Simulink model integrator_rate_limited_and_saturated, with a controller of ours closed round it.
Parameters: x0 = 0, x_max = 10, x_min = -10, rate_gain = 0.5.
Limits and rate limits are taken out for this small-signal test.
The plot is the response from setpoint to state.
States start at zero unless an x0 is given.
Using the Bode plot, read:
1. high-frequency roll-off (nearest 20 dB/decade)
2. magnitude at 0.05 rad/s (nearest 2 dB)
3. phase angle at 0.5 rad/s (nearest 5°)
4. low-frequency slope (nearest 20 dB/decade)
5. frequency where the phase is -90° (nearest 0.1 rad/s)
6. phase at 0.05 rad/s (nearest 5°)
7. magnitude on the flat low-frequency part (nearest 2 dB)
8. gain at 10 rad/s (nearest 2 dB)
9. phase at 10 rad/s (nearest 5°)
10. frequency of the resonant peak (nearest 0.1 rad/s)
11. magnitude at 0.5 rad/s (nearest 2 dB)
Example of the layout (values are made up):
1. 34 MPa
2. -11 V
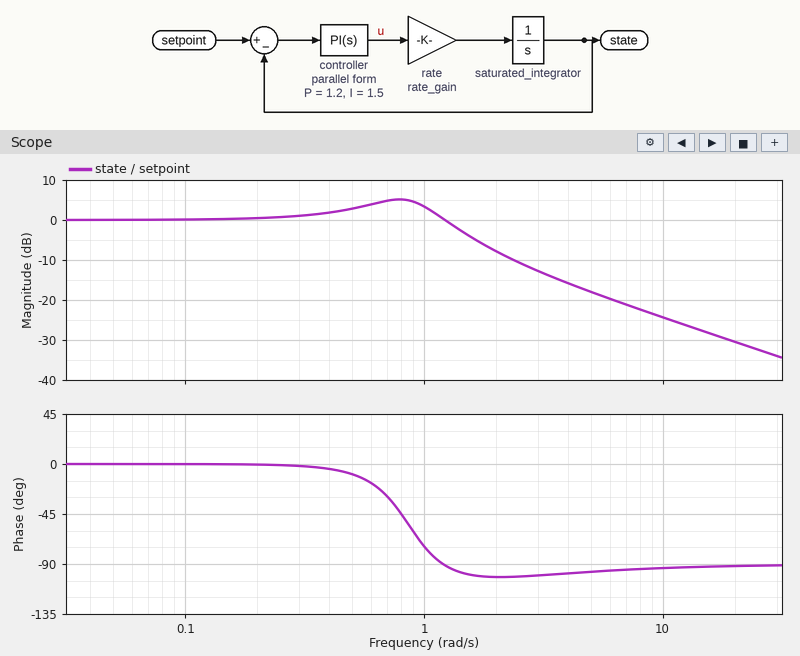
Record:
1. -20 dB/decade
2. 0 dB
3. -10°
4. 0 dB/decade
5. 1.2 rad/s
6. 0°
7. 0 dB
8. -24 dB
9. -95°
10. 0.8 rad/s
11. 2 dB
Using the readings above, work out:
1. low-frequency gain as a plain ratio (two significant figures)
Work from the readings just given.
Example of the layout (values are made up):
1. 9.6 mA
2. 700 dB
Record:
1. 1.0
